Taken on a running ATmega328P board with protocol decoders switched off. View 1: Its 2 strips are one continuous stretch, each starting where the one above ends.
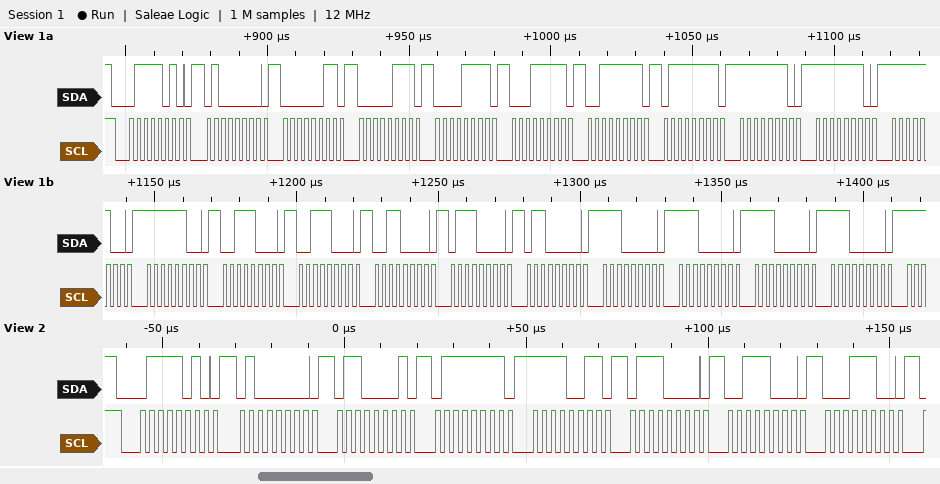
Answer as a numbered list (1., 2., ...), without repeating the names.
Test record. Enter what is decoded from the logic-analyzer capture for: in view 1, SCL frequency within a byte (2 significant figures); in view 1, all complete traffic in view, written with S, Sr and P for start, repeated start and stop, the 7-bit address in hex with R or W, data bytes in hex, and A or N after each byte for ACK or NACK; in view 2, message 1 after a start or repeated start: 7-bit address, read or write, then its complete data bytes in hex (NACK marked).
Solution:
1. 400 kHz
2. S 3DW A 40 A 03 A 07 A 0F A 1F A 3F A 7F A FE A FE A FC A FC A 38 A 38 A 30 A 70 A 60 A E0 A E0 A E0 A E0 A
3. 0x3D write: 40 61 7F F3 70 38 1C
